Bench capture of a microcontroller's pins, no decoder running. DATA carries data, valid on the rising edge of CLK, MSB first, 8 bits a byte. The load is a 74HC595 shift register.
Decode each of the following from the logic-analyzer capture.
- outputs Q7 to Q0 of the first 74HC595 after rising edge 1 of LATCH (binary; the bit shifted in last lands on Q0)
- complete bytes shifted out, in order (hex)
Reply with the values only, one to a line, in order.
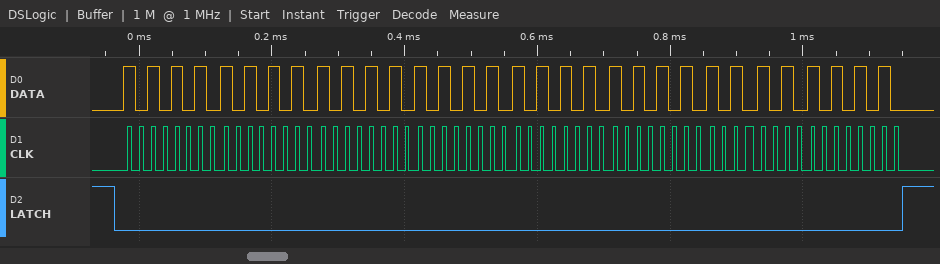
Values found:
10101010
0xAA 0xAA 0xAA 0xAA 0xAA 0xAA 0xAA 0xAA
